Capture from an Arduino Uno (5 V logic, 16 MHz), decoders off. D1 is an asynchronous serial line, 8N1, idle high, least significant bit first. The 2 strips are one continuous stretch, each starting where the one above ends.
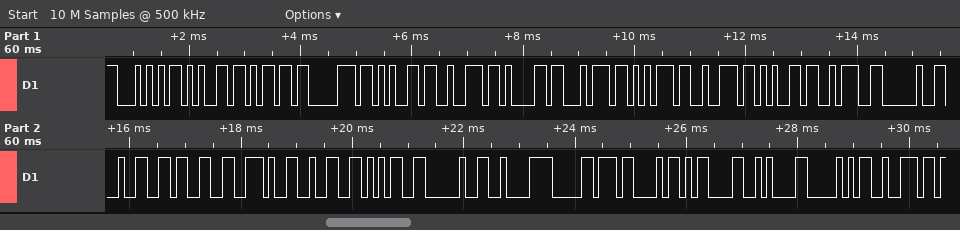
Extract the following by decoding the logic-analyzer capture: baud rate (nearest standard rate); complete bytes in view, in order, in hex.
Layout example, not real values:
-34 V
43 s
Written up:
9600 baud
54 65 6D 70 65 72 61 74 75 72 65 3A 20 32 33 2E 32 35 20 C2 B0 43 0D 0A 50 72
